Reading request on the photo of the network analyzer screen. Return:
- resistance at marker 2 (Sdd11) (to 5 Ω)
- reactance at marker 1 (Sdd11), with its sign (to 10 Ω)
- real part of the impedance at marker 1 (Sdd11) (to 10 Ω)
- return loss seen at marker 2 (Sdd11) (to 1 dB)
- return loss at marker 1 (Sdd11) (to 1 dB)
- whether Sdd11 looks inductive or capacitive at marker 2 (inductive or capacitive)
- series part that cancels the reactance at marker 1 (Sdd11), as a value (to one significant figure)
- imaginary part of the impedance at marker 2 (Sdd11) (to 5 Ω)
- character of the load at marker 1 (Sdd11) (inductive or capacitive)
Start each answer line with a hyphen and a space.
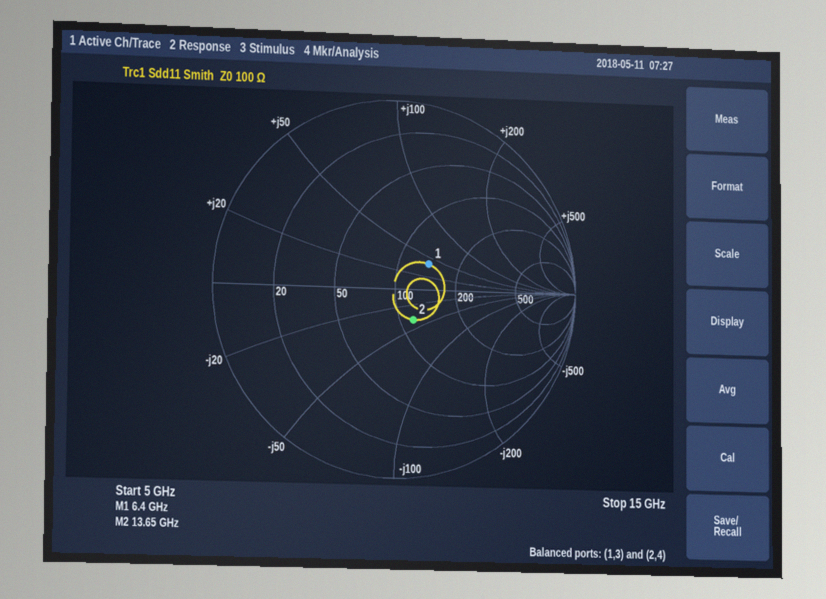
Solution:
- 115 Ω
- +40 Ω
- 140 Ω
- 14 dB
- 13 dB
- capacitive
- 600 fF
- -40 Ω
- inductive
